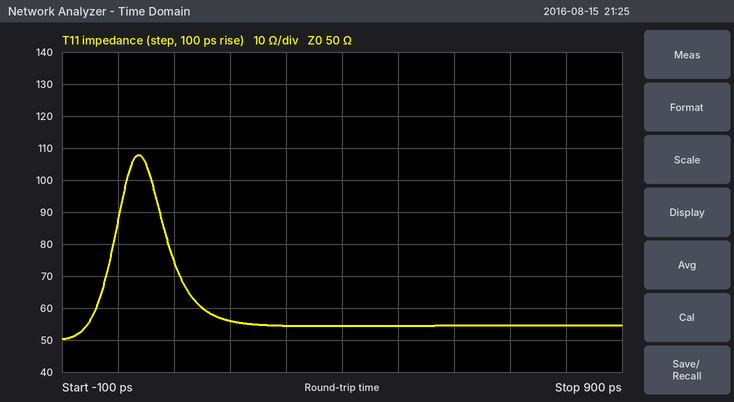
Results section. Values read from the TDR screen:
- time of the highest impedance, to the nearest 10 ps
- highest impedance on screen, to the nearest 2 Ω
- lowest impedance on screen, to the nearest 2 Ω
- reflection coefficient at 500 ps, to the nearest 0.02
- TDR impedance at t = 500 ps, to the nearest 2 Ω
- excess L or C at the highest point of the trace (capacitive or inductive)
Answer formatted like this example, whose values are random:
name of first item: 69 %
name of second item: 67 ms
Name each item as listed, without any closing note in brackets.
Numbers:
time of the highest impedance, to the nearest 10 ps: 40 ps
highest impedance on screen, to the nearest 2 Ω: 108 Ω
lowest impedance on screen, to the nearest 2 Ω: 50 Ω
reflection coefficient at 500 ps, to the nearest 0.02: +0.04
TDR impedance at t = 500 ps, to the nearest 2 Ω: 54 Ω
excess L or C at the highest point of the trace: inductive
